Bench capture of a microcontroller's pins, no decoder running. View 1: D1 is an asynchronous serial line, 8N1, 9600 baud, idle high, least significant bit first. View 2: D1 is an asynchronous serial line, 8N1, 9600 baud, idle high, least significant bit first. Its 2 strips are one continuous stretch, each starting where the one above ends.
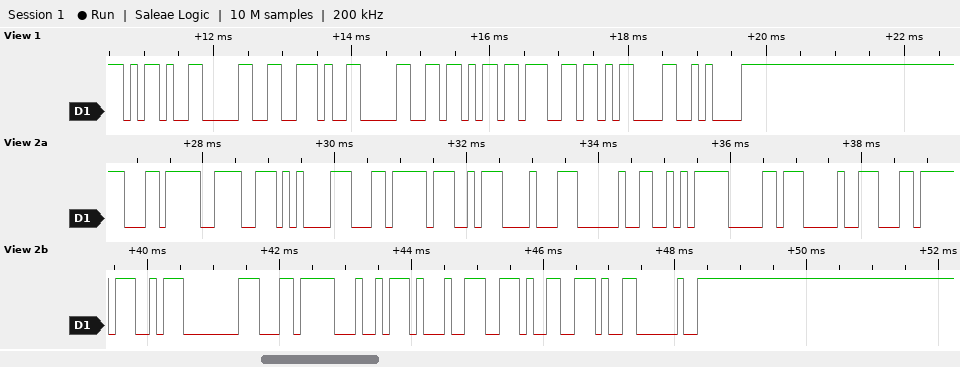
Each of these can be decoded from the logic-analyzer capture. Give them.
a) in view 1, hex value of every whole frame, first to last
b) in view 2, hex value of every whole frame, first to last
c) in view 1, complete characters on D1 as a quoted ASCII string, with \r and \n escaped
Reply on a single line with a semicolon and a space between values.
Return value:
2D 30 2E 30 6B 67 0D 0A; EC 9E 85 EC A7 88 20 EA B0 90 EC A7 80 EC A4 91 2E 2E 20; "-0.0kg\r\n"
